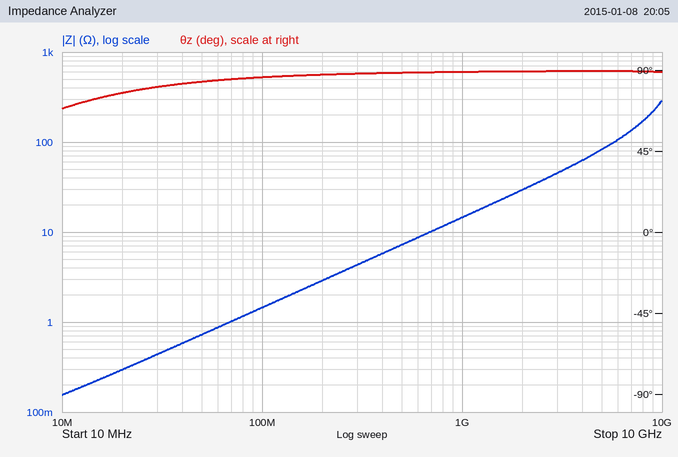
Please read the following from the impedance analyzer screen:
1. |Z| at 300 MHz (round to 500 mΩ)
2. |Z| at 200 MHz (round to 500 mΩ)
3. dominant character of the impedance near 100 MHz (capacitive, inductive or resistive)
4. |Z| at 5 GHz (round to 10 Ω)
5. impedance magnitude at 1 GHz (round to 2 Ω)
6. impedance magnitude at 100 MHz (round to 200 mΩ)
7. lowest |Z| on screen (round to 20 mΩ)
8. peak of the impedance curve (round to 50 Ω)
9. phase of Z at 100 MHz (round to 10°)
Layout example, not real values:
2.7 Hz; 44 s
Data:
4.5 Ω; 3.0 Ω; inductive; 80 Ω; 14 Ω; 1.4 Ω; 160 mΩ; 300 Ω; 90°
